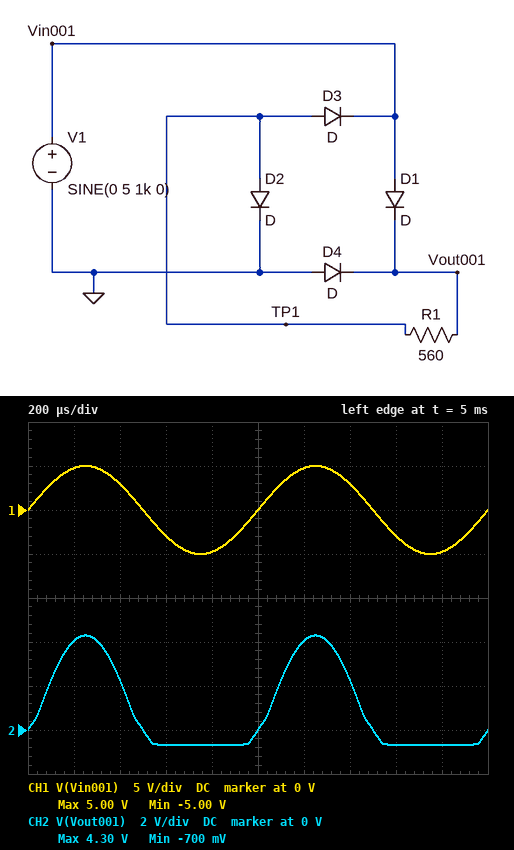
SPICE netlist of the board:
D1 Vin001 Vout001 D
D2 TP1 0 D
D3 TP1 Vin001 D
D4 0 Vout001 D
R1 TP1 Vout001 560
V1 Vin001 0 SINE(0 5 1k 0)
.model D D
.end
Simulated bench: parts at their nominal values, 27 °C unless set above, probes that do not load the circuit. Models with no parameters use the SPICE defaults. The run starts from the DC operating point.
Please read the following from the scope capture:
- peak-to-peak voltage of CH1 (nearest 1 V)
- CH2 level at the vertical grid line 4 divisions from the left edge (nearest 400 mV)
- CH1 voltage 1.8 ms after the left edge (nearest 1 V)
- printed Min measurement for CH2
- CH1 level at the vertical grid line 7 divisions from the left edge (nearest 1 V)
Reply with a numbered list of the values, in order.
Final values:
1. 10 V
2. -800 mV
3. -5 V
4. -700 mV
5. 3 V
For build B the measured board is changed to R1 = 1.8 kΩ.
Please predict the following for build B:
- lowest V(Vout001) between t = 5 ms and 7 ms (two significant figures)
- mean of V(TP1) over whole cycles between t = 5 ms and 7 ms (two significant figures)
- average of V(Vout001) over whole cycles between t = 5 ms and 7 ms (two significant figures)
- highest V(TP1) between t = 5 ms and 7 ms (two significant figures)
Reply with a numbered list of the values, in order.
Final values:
1. -670 mV
2. -990 mV
3. 990 mV
4. 670 mV
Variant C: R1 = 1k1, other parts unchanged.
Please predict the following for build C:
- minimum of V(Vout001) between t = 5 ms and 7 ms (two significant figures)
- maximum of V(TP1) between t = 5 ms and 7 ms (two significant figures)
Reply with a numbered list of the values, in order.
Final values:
1. -690 mV
2. 690 mV
